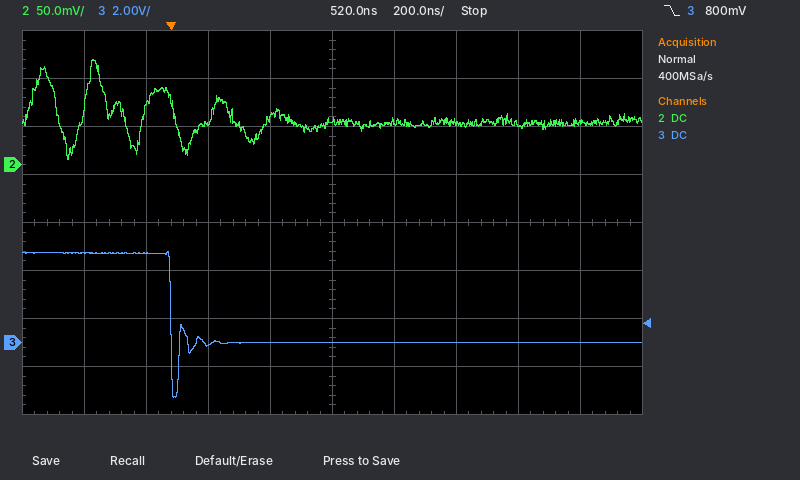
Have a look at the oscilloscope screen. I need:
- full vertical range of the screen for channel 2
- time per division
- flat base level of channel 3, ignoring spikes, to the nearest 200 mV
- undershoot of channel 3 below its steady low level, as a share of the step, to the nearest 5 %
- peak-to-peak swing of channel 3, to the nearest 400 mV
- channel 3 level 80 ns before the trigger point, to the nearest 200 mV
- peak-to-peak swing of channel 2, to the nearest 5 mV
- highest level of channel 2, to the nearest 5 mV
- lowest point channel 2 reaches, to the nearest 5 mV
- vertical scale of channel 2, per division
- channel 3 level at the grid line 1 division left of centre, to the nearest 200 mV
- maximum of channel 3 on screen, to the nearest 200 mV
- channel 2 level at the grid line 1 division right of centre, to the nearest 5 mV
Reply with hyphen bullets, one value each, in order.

- 400 mV
- 200 ns
- 0.0 V
- 60 %
- 6.0 V
- 3.8 V
- 105 mV
- 110 mV
- 5 mV
- 50 mV
- 0.0 V
- 3.8 V
- 45 mV
